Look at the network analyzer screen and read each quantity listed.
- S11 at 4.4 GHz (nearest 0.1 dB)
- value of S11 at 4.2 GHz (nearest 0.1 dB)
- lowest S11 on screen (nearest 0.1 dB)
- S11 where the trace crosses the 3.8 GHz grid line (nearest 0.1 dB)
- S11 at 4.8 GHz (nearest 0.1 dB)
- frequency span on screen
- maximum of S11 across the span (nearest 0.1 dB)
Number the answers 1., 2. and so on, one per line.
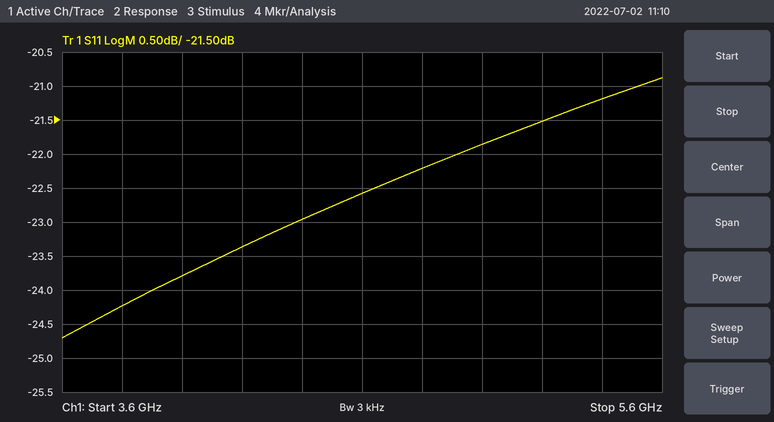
1. -23.0 dB
2. -23.4 dB
3. -24.7 dB
4. -24.2 dB
5. -22.2 dB
6. 2 GHz
7. -20.9 dB
